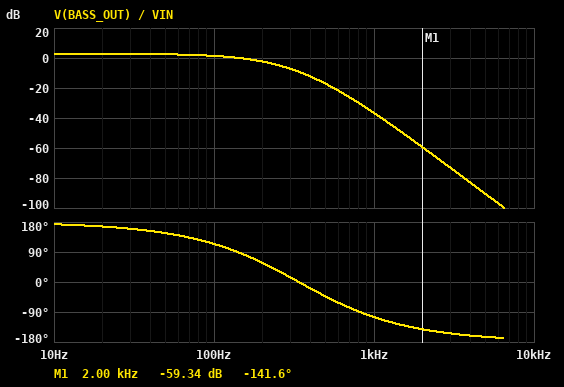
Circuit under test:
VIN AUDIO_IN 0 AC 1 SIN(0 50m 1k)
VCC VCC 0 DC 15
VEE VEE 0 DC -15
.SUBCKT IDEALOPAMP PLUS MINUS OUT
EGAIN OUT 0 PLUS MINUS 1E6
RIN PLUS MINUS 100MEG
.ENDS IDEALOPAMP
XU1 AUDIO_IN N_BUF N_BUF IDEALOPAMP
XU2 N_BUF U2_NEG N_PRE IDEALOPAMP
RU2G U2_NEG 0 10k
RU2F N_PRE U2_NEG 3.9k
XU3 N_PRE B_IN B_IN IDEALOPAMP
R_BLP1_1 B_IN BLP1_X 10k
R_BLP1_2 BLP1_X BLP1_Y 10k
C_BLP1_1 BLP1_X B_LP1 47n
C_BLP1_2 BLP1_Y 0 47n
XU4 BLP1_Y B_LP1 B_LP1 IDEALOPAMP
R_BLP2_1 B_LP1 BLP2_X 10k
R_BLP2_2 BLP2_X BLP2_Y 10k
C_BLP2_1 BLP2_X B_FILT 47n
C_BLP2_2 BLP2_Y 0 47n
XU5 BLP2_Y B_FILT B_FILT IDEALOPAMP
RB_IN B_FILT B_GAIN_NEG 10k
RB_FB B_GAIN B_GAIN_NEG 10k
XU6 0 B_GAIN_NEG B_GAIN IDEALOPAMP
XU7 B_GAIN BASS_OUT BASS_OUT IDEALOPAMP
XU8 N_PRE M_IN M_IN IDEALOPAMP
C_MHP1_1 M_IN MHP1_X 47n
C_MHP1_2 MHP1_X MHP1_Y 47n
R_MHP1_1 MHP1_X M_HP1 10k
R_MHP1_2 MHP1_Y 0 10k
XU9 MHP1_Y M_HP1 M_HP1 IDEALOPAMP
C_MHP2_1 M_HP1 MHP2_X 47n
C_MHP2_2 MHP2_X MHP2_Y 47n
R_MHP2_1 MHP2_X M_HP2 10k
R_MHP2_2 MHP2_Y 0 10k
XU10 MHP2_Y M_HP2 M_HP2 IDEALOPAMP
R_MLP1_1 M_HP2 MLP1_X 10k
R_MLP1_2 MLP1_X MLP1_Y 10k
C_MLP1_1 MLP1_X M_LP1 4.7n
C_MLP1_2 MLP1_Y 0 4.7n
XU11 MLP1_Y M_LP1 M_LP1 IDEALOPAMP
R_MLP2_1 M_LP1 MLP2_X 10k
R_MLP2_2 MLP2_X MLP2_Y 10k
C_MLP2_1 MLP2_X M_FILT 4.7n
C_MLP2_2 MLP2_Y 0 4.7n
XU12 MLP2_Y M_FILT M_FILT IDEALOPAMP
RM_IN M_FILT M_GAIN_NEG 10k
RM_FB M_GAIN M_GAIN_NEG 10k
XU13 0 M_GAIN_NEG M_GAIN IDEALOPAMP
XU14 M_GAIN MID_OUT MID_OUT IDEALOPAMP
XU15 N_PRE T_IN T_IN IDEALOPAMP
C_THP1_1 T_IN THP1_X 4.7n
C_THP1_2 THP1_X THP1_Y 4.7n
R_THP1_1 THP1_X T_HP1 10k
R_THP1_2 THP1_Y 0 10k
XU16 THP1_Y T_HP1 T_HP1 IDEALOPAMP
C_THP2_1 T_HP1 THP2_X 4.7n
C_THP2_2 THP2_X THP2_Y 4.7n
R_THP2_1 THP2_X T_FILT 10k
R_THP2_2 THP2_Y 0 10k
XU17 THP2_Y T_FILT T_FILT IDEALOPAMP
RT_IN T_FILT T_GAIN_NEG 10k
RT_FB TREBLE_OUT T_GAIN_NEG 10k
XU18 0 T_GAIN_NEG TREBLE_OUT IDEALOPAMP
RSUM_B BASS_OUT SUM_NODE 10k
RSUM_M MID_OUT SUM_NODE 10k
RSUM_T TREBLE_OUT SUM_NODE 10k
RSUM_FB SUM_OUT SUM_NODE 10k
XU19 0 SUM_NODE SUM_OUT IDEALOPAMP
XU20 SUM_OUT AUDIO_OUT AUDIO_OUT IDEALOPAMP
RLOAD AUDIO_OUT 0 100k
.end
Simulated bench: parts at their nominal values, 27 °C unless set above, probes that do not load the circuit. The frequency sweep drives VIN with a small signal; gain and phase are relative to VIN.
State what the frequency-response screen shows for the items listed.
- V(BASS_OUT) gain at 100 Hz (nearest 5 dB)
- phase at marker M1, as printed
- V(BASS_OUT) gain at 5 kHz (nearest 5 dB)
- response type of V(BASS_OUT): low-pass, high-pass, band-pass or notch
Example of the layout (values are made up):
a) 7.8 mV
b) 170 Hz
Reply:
a) 0 dB
b) -141.6 deg
c) -90 dB
d) low-pass
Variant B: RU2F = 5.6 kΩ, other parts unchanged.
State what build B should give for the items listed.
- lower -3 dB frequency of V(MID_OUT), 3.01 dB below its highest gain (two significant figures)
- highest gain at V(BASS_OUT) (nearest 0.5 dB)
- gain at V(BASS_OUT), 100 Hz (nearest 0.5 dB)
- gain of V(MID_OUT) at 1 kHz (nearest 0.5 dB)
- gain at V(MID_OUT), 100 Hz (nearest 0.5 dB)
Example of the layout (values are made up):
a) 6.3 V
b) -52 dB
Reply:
a) 530 Hz
b) 4.0 dB
c) 2.5 dB
d) 0.5 dB
e) -40.0 dB
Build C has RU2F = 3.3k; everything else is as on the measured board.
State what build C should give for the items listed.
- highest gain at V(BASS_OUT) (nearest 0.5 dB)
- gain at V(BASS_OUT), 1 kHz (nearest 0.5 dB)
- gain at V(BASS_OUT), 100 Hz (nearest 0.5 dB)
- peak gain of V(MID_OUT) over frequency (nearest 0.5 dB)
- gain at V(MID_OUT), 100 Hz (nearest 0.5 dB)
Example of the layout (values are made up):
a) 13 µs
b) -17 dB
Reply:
a) 2.5 dB
b) -37.0 dB
c) 1.0 dB
d) -1.0 dB
e) -41.5 dB
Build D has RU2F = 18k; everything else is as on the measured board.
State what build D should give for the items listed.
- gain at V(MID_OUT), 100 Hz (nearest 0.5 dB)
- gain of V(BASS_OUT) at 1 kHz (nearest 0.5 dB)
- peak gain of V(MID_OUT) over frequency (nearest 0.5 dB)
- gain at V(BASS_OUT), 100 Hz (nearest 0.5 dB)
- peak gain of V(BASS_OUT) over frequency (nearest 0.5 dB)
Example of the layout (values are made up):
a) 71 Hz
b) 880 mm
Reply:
a) -35.0 dB
b) -30.5 dB
c) 5.5 dB
d) 7.5 dB
e) 9.0 dB
